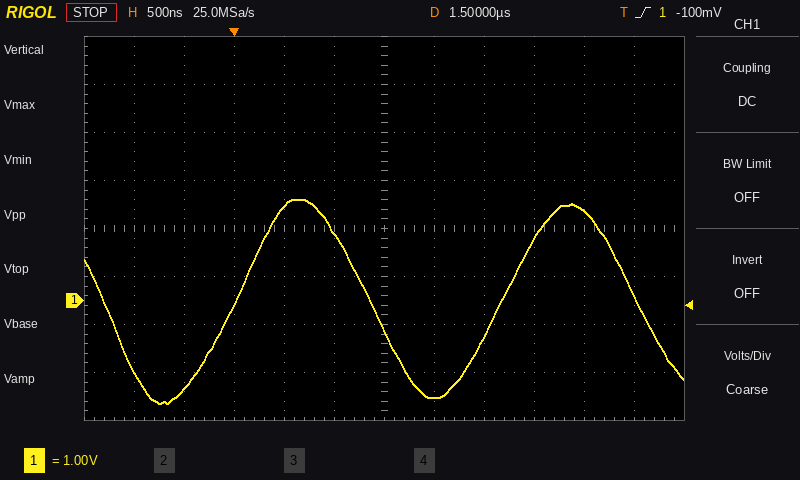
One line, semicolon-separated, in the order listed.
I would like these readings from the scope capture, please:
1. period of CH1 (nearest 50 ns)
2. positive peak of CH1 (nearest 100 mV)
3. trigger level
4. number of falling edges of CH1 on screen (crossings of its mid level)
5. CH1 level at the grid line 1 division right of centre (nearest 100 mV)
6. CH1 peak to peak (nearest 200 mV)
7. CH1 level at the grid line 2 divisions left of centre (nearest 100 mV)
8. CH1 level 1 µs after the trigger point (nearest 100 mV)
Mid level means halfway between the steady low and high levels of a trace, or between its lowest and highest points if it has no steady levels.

2.65 µs; 2.1 V; -100 mV; 3; -2.0 V; 4.2 V; 2.0 V; 1.4 V
